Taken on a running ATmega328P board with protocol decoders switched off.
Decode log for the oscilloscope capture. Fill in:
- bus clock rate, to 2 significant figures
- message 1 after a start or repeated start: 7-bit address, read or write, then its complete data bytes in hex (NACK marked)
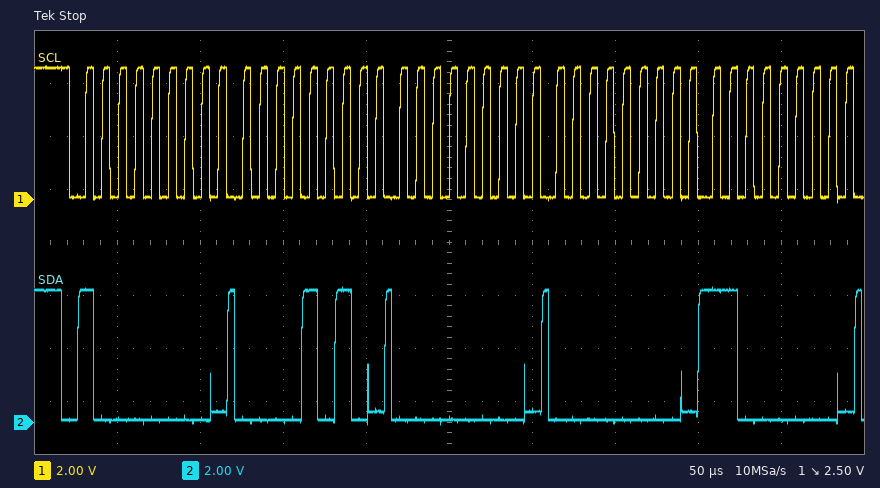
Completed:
100 kHz
0x40 write: 0A 00 00 C0
